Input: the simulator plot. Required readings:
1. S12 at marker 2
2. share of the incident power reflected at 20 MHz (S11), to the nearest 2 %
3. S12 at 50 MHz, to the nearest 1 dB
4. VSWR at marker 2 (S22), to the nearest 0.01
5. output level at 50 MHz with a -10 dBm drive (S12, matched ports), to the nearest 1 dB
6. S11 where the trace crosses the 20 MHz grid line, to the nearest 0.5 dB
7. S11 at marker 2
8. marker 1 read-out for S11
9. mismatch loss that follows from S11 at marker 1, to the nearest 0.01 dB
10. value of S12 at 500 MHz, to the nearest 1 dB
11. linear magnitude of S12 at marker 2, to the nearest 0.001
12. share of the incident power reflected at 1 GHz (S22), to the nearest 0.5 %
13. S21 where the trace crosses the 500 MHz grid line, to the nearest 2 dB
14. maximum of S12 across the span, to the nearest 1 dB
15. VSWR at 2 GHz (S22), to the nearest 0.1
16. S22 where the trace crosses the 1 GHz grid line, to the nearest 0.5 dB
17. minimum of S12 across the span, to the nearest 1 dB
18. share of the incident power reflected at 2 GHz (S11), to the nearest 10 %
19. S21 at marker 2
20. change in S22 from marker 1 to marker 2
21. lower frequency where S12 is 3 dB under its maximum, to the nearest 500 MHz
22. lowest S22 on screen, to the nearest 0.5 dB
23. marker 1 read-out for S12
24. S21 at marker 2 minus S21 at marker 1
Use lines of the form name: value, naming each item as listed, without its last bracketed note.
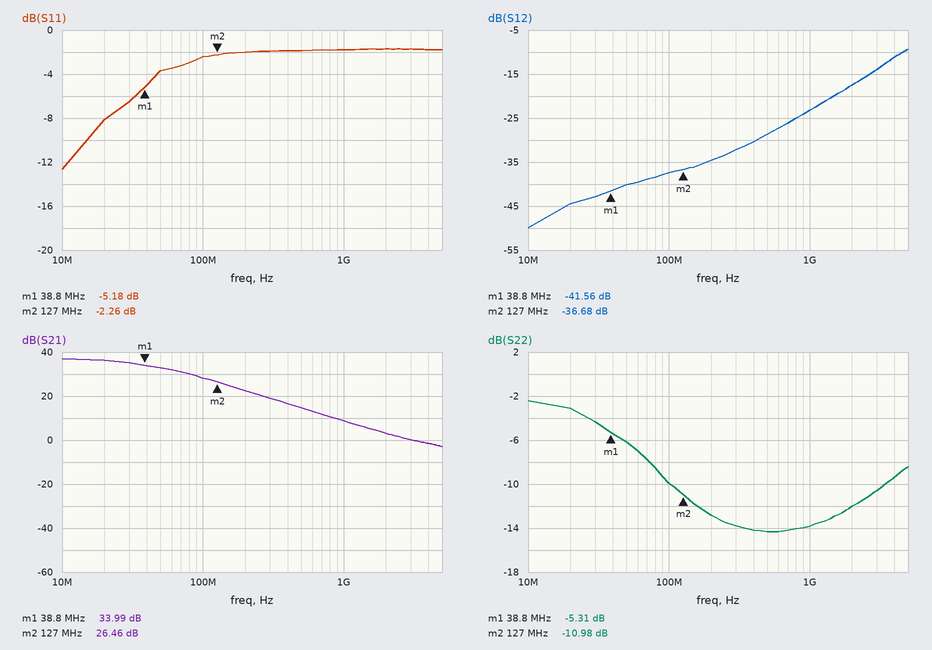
S12 at marker 2: -36.68 dB
share of the incident power reflected at 20 MHz (S11), to the nearest 2 %: 16 %
S12 at 50 MHz, to the nearest 1 dB: -40 dB
VSWR at marker 2 (S22), to the nearest 0.01: 1.79
output level at 50 MHz with a -10 dBm drive (S12, matched ports), to the nearest 1 dB: -50 dBm
S11 where the trace crosses the 20 MHz grid line, to the nearest 0.5 dB: -8.0 dB
S11 at marker 2: -2.26 dB
marker 1 read-out for S11: -5.18 dB
mismatch loss that follows from S11 at marker 1, to the nearest 0.01 dB: 1.57 dB
value of S12 at 500 MHz, to the nearest 1 dB: -29 dB
linear magnitude of S12 at marker 2, to the nearest 0.001: 0.015
share of the incident power reflected at 1 GHz (S22), to the nearest 0.5 %: 4.0 %
S21 where the trace crosses the 500 MHz grid line, to the nearest 2 dB: 14 dB
maximum of S12 across the span, to the nearest 1 dB: -9 dB
VSWR at 2 GHz (S22), to the nearest 0.1: 1.7
S22 where the trace crosses the 1 GHz grid line, to the nearest 0.5 dB: -14.0 dB
minimum of S12 across the span, to the nearest 1 dB: -50 dB
share of the incident power reflected at 2 GHz (S11), to the nearest 10 %: 70 %
S21 at marker 2: 26.46 dB
change in S22 from marker 1 to marker 2: -5.67 dB
lower frequency where S12 is 3 dB under its maximum, to the nearest 500 MHz: 3.5 GHz
lowest S22 on screen, to the nearest 0.5 dB: -14.5 dB
marker 1 read-out for S12: -41.56 dB
S21 at marker 2 minus S21 at marker 1: -7.53 dB
